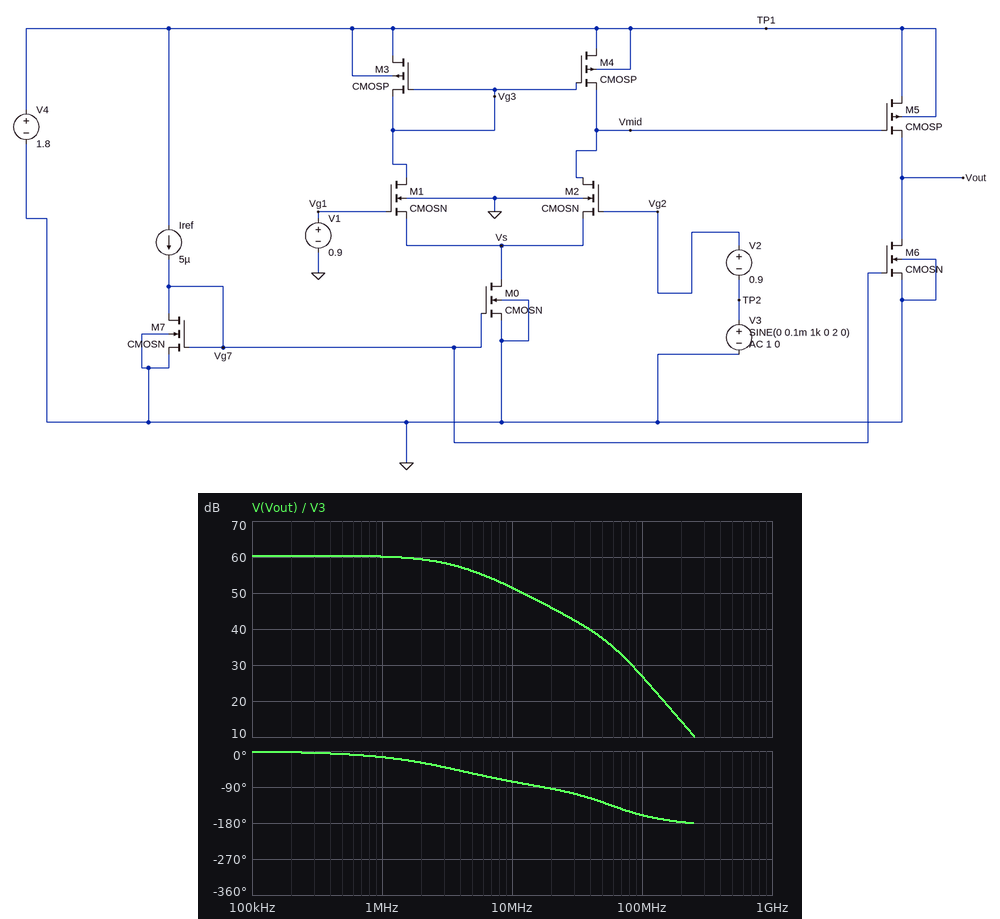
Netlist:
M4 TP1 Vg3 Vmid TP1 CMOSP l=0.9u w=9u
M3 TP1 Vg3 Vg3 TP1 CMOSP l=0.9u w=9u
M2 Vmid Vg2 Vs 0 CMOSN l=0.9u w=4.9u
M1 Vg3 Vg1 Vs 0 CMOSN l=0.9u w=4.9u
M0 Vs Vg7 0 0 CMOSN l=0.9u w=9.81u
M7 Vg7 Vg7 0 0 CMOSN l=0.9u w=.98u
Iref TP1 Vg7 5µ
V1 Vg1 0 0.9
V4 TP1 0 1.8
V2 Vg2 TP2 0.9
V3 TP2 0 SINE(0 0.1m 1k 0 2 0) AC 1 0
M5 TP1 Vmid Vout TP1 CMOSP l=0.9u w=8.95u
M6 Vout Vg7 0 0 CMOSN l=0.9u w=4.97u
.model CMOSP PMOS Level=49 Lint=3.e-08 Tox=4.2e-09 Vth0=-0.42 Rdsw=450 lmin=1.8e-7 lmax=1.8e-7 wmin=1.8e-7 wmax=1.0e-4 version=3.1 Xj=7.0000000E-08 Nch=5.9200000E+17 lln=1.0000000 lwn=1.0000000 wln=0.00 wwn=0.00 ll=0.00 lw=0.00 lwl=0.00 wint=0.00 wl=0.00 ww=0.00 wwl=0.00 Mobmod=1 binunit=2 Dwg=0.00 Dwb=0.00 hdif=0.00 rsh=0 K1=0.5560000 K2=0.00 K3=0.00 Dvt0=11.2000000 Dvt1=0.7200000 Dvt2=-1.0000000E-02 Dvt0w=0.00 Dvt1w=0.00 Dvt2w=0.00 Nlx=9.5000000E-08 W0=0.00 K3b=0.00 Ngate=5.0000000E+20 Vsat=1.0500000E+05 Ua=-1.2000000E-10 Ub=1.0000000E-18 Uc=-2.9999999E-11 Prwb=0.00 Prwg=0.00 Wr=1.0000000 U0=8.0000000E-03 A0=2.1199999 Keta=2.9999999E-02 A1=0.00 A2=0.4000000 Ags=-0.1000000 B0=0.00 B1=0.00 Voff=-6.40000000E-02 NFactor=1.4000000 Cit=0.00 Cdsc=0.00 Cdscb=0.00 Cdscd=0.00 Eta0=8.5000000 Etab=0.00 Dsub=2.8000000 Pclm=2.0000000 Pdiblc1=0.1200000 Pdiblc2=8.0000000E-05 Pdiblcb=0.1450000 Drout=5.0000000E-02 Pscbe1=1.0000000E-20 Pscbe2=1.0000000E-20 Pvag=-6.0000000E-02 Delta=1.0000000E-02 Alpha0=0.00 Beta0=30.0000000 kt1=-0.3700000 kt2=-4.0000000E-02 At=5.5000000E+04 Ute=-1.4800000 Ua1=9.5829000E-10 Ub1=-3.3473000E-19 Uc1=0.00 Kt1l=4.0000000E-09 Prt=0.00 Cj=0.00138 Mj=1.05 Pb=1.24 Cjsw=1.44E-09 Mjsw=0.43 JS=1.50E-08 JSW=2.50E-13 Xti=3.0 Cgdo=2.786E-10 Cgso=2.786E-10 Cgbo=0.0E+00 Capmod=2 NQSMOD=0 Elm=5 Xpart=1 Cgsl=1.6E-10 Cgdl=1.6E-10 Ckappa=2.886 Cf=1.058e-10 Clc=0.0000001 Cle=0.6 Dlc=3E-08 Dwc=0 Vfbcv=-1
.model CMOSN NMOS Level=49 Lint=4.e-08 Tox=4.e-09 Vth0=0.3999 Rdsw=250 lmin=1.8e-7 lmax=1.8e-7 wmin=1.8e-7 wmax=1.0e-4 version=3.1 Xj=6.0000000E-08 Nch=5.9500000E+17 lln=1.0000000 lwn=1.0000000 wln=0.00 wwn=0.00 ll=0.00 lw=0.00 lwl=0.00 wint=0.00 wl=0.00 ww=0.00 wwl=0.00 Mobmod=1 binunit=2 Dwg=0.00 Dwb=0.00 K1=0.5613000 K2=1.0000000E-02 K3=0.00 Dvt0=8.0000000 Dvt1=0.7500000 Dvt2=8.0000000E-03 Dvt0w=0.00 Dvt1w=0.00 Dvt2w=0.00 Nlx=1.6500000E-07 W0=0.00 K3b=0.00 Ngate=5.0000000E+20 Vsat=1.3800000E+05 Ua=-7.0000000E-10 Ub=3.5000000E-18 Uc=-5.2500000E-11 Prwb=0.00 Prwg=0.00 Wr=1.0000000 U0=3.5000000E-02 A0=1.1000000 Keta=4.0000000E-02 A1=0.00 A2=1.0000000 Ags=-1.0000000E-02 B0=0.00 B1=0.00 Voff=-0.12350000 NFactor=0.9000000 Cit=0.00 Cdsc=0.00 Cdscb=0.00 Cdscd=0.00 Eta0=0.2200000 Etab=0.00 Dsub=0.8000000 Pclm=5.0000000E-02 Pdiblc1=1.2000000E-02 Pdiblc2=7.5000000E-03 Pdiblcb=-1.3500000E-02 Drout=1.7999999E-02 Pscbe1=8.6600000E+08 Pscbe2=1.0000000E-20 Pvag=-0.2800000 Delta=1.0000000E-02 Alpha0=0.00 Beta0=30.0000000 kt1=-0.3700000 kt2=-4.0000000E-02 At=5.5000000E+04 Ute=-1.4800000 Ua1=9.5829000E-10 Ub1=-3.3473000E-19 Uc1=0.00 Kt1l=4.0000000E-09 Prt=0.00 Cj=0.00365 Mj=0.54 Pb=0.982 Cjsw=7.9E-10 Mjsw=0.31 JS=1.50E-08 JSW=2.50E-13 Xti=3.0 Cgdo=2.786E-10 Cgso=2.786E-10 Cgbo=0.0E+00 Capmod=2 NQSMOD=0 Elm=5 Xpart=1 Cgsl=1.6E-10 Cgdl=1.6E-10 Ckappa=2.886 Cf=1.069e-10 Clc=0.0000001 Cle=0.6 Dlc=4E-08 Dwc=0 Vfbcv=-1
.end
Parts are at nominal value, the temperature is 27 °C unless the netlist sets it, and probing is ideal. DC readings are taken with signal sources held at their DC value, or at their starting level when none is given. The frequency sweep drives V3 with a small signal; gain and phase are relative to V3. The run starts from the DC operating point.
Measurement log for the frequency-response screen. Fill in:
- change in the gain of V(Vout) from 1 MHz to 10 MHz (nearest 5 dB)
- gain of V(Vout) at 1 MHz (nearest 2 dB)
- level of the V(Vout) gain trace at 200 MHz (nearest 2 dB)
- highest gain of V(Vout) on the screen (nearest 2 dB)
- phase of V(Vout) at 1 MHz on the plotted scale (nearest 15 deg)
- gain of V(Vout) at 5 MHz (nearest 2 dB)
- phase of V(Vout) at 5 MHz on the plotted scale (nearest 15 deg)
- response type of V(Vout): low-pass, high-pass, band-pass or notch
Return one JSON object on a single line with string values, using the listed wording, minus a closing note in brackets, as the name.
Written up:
{"change in the gain of V(Vout) from 1 MHz to 10 MHz": "-10 dB", "gain of V(Vout) at 1 MHz": "60 dB", "level of the V(Vout) gain trace at 200 MHz": "14 dB", "highest gain of V(Vout) on the screen": "60 dB", "phase of V(Vout) at 1 MHz on the plotted scale": "-15 deg", "gain of V(Vout) at 5 MHz": "56 dB", "phase of V(Vout) at 5 MHz on the plotted scale": "-60 deg", "response type of V(Vout): low-pass, high-pass, band-pass or notch": "low-pass"}
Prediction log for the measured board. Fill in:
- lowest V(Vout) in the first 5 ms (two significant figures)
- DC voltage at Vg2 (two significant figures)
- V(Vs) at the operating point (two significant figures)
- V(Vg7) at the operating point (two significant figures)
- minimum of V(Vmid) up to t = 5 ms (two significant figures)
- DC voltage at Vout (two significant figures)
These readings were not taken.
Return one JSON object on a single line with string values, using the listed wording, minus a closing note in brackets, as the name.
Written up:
{"lowest V(Vout) in the first 5 ms": "420 mV", "DC voltage at Vg2": "900 mV", "V(Vs) at the operating point": "220 mV", "V(Vg7) at the operating point": "620 mV", "minimum of V(Vmid) up to t = 5 ms": "1.0 V", "DC voltage at Vout": "530 mV"}
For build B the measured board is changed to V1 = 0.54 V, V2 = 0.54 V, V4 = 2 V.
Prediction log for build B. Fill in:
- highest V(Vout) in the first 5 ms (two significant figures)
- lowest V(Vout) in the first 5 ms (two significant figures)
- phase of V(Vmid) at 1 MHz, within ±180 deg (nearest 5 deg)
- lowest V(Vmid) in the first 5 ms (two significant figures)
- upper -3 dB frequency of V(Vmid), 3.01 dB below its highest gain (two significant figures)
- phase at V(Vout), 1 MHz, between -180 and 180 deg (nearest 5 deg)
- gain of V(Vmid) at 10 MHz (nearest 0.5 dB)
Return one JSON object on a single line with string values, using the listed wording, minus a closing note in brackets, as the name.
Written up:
{"highest V(Vout) in the first 5 ms": "35 mV", "lowest V(Vout) in the first 5 ms": "30 mV", "phase of V(Vmid) at 1 MHz, within ±180 deg": "160 deg", "lowest V(Vmid) in the first 5 ms": "1.4 V", "upper -3 dB frequency of V(Vmid), 3.01 dB below its highest gain": "3.0 MHz", "phase at V(Vout), 1 MHz, between -180 and 180 deg": "-20 deg", "gain of V(Vmid) at 10 MHz": "24.5 dB"}
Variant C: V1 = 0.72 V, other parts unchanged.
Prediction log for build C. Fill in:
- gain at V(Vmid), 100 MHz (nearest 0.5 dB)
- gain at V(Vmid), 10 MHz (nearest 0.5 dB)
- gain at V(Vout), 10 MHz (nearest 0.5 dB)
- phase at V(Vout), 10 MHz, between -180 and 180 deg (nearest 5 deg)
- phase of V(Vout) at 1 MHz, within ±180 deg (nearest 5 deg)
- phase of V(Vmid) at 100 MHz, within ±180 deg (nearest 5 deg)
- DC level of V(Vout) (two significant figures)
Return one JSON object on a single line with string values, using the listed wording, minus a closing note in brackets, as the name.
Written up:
{"gain at V(Vmid), 100 MHz": "-14.5 dB", "gain at V(Vmid), 10 MHz": "-15.5 dB", "gain at V(Vout), 10 MHz": "-46.0 dB", "phase at V(Vout), 10 MHz, between -180 and 180 deg": "-10 deg", "phase of V(Vout) at 1 MHz, within ±180 deg": "0 deg", "phase of V(Vmid) at 100 MHz, within ±180 deg": "145 deg", "DC level of V(Vout)": "1.8 V"}
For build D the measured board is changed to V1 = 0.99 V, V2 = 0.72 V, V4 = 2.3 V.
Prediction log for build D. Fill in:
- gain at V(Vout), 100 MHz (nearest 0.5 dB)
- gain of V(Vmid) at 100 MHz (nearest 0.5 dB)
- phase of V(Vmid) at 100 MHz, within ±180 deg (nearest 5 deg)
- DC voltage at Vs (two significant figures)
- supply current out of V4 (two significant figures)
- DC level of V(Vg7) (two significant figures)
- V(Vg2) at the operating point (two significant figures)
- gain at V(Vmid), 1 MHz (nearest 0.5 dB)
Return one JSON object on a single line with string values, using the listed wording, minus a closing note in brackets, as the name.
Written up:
{"gain at V(Vout), 100 MHz": "-60.5 dB", "gain of V(Vmid) at 100 MHz": "-19.5 dB", "phase of V(Vmid) at 100 MHz, within ±180 deg": "155 deg", "DC voltage at Vs": "230 mV", "supply current out of V4": "52 µA", "DC level of V(Vg7)": "620 mV", "V(Vg2) at the operating point": "720 mV", "gain at V(Vmid), 1 MHz": "-19.0 dB"}
